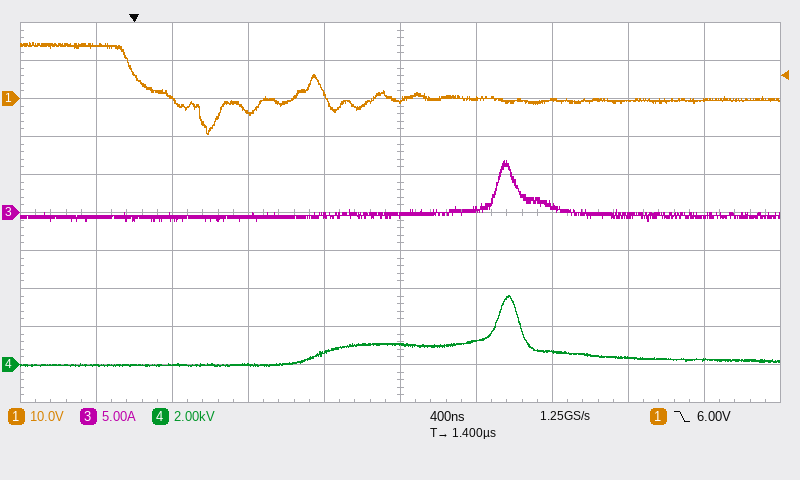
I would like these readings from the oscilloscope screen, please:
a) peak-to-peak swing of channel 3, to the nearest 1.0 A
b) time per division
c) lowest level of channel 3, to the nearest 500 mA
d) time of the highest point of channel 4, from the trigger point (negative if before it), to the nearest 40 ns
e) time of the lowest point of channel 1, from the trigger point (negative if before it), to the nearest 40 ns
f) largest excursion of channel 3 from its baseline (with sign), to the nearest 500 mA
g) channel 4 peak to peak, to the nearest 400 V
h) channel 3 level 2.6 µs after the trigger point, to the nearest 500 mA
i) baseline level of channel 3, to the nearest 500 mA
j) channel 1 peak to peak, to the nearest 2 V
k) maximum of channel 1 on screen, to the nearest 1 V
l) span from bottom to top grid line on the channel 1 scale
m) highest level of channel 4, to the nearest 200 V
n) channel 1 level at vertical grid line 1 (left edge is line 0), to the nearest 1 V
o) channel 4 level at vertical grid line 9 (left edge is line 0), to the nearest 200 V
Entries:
8.0 A
400 ns
-1.0 A
+1.96 µs
+400 ns
+7.5 A
3.6 kV
-500 mA
-500 mA
24 V
15 V
100 V
3.6 kV
14 V
200 V
